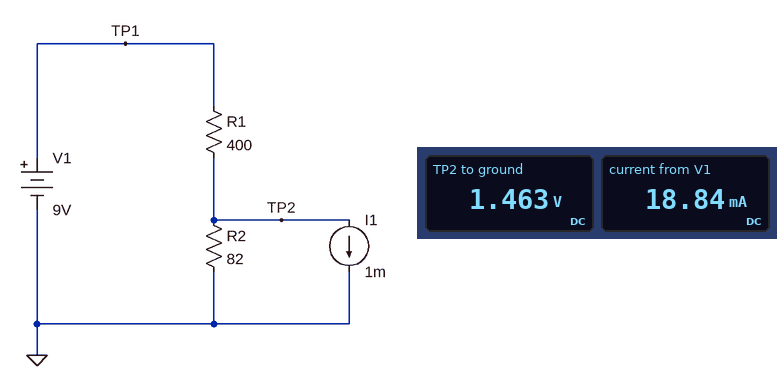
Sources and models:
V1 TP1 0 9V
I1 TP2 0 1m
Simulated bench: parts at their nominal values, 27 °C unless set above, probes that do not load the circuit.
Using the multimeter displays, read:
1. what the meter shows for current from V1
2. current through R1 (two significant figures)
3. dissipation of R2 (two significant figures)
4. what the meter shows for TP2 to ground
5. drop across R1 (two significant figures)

18.84 mA
19 mA
26 mW
1.463 V
7.5 V
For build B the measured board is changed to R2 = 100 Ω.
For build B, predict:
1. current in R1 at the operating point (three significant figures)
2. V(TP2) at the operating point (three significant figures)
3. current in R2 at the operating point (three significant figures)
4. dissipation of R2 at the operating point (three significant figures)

18.2 mA
1.72 V
17.2 mA
29.6 mW
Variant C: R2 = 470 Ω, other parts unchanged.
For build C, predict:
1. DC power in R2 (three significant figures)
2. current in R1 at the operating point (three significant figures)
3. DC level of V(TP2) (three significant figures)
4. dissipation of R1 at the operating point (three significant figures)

45.9 mW
10.9 mA
4.65 V
47.4 mW
